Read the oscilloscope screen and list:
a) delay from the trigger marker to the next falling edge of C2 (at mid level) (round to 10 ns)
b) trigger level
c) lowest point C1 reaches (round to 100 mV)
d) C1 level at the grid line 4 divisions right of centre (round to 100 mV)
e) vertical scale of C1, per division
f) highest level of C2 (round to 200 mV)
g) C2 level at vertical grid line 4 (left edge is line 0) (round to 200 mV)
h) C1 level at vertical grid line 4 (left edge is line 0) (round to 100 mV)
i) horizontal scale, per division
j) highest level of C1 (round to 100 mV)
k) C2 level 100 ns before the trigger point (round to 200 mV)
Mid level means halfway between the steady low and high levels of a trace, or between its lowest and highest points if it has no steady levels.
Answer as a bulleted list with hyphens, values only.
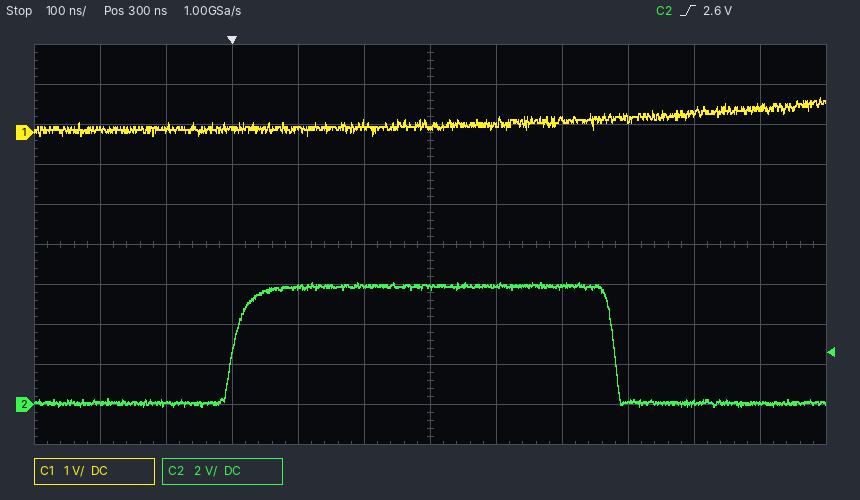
- 580 ns
- 2.6 V
- -100 mV
- 500 mV
- 1 V
- 6.0 V
- 5.8 V
- 100 mV
- 100 ns
- 900 mV
- 0.0 V
